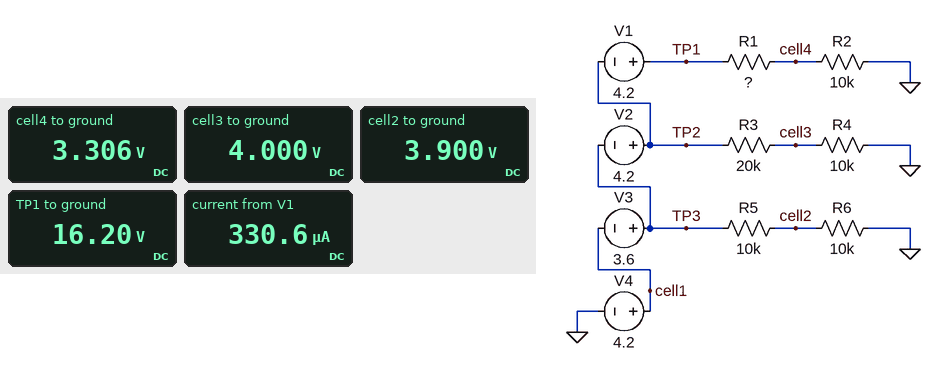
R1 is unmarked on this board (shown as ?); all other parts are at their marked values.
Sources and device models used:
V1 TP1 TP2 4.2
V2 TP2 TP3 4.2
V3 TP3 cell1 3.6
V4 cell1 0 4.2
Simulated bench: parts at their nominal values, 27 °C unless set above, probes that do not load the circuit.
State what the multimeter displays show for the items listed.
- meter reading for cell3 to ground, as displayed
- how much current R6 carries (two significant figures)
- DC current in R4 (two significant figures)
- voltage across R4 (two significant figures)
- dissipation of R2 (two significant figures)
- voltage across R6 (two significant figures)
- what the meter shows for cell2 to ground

4.000 V
390 µA
400 µA
4.0 V
1.1 mW
3.9 V
3.900 V
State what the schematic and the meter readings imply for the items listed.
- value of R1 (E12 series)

39 kΩ
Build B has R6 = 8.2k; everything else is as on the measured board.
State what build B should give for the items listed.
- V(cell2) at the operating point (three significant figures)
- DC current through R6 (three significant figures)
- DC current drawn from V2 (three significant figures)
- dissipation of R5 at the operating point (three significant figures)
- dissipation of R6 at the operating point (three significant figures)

3.51 V
429 µA
731 µA
1.84 mW
1.51 mW
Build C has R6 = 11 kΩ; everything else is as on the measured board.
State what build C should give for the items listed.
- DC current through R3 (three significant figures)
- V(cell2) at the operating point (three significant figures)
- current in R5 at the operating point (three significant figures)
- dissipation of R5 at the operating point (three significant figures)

400 µA
4.09 V
371 µA
1.38 mW
